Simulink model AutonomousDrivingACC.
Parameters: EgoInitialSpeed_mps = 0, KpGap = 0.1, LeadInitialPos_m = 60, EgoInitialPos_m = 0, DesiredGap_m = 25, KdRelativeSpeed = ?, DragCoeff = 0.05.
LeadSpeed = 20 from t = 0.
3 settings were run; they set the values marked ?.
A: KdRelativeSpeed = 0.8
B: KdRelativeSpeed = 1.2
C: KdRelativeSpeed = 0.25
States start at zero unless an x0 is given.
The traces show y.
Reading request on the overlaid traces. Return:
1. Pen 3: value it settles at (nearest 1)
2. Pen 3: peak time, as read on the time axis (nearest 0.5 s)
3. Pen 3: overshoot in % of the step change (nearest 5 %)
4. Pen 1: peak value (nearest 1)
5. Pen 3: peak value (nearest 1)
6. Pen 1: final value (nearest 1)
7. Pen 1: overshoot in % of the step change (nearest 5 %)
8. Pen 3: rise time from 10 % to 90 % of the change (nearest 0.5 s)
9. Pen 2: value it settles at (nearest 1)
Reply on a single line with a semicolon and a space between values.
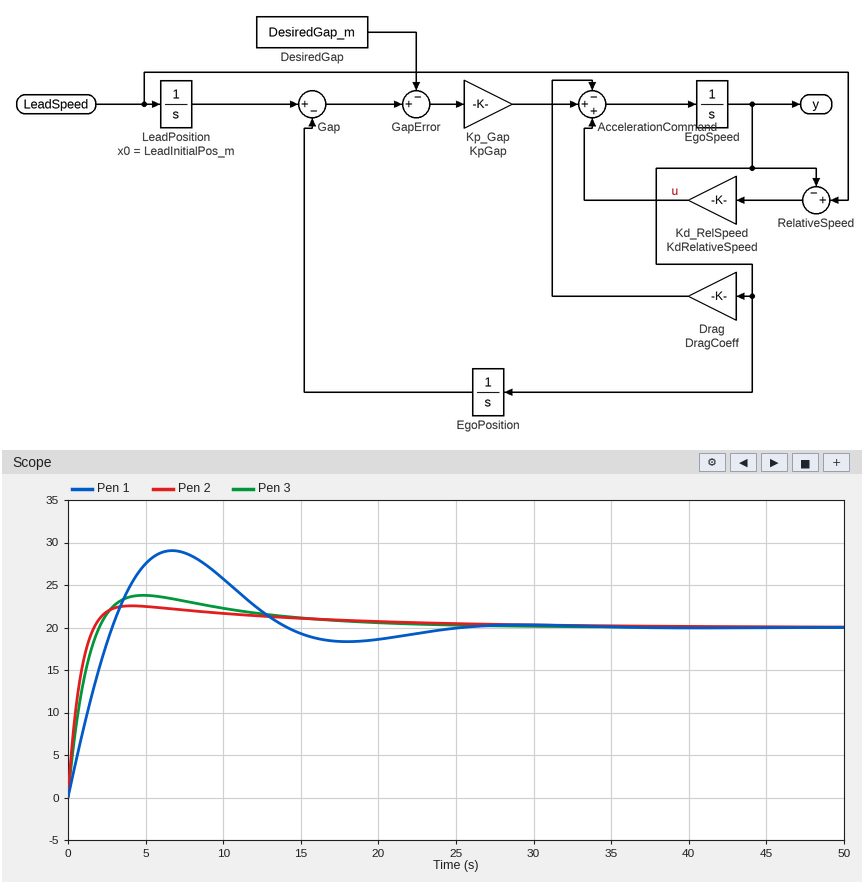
20; 5.0 s; 20 %; 29; 24; 20; 45 %; 1.5 s; 20
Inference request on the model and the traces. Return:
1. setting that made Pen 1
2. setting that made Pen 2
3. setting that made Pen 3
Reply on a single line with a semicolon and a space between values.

C; B; A
